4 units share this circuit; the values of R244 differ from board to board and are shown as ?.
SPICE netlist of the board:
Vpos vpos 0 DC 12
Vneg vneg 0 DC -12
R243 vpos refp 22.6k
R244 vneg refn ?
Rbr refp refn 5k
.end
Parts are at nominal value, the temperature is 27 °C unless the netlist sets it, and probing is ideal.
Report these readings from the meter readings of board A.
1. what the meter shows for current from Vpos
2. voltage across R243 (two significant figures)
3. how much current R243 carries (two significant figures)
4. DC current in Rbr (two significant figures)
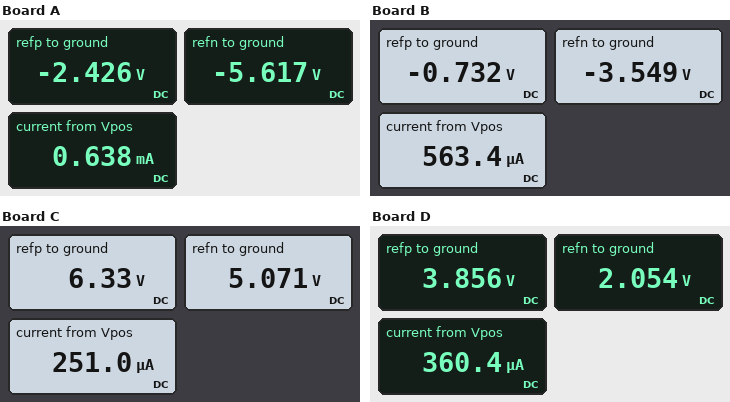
0.638 mA
14 V
640 µA
640 µA
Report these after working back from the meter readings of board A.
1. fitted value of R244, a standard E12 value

10 kΩ
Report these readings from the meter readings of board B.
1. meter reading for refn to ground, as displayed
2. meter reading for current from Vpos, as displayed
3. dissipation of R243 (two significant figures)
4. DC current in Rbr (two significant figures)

-3.549 V
563.4 µA
7.2 mW
560 µA
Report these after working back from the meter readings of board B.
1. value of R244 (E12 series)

15 kΩ
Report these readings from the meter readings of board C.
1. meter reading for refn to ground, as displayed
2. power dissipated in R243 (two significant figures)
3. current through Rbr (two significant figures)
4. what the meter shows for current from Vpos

5.071 V
1.4 mW
250 µA
251.0 µA
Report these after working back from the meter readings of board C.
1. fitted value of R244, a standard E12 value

68 kΩ
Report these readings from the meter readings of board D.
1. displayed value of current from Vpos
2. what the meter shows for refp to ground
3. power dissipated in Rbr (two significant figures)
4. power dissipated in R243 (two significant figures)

360.4 µA
3.856 V
650 µW
2.9 mW
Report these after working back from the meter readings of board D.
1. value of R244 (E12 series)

39 kΩ
